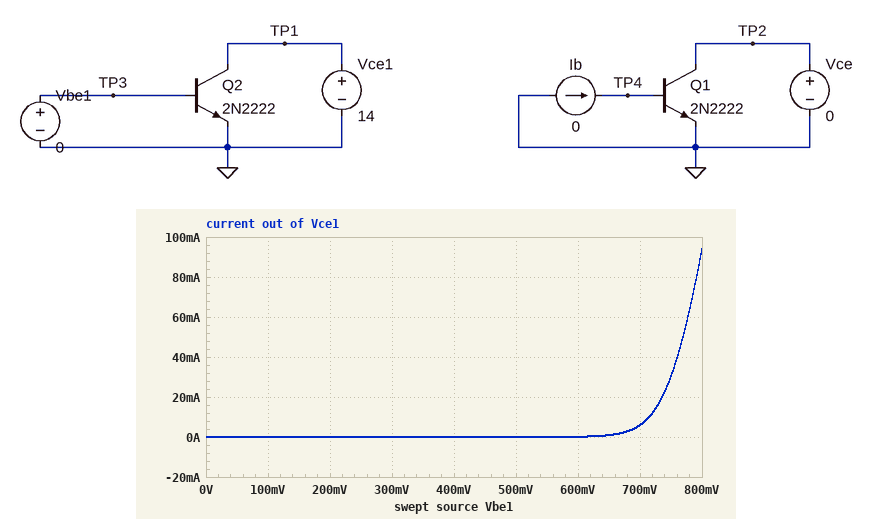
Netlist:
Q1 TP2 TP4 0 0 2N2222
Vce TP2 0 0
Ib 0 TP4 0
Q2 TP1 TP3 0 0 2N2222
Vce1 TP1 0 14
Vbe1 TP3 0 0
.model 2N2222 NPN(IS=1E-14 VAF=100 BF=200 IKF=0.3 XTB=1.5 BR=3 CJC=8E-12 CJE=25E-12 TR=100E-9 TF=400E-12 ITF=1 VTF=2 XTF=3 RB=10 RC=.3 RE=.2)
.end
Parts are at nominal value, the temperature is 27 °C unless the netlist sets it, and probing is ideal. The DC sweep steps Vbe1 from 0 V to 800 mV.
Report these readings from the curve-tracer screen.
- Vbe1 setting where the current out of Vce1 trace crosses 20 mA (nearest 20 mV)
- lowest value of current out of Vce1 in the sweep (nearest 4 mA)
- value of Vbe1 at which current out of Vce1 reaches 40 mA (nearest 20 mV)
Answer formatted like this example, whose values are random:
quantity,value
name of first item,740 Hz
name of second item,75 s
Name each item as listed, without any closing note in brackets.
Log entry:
quantity,value
Vbe1 setting where the current out of Vce1 trace crosses 20 mA,740 mV
lowest value of current out of Vce1 in the sweep,0 A
value of Vbe1 at which current out of Vce1 reaches 40 mA,760 mV
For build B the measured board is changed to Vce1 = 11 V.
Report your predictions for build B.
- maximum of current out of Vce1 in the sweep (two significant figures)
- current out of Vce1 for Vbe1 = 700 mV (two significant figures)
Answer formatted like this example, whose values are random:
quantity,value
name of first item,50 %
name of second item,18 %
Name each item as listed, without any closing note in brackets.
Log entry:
quantity,value
maximum of current out of Vce1 in the sweep,92 mA
current out of Vce1 for Vbe1 = 700 mV,5.8 mA
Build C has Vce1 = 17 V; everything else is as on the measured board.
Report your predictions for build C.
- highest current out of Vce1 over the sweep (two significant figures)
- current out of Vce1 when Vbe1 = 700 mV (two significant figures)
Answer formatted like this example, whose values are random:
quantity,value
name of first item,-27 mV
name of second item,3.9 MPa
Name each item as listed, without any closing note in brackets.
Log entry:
quantity,value
highest current out of Vce1 over the sweep,96 mA
current out of Vce1 when Vbe1 = 700 mV,6.1 mA
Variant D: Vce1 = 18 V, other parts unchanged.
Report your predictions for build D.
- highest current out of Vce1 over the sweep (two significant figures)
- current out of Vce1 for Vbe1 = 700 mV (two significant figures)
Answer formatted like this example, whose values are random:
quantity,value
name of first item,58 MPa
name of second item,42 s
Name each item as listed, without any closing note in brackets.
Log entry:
quantity,value
highest current out of Vce1 over the sweep,96 mA
current out of Vce1 for Vbe1 = 700 mV,6.2 mA
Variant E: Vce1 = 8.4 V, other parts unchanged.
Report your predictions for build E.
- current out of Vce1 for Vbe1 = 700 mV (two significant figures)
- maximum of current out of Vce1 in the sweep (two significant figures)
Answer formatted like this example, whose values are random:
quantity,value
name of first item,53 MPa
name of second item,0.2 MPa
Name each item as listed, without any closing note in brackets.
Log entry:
quantity,value
current out of Vce1 for Vbe1 = 700 mV,5.7 mA
maximum of current out of Vce1 in the sweep,91 mA
